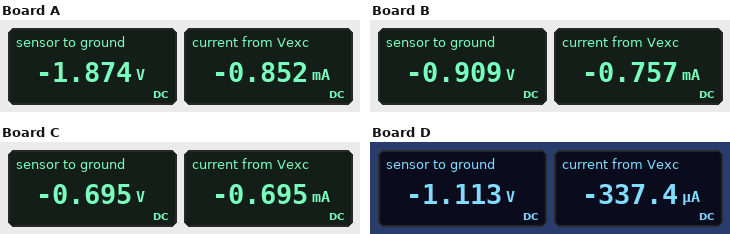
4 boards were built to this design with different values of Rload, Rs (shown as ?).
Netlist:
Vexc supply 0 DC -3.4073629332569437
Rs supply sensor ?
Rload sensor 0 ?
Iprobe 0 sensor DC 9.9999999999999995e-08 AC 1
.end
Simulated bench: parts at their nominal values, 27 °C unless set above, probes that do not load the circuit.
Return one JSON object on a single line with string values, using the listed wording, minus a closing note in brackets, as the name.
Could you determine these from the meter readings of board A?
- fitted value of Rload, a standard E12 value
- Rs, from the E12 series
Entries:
{"fitted value of Rload, a standard E12 value": "2.2 kΩ", "Rs, from the E12 series": "1.8 kΩ"}
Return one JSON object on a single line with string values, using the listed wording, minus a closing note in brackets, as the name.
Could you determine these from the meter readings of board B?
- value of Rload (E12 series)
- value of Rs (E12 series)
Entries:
{"value of Rload": "1.2 kΩ", "value of Rs": "3.3 kΩ"}
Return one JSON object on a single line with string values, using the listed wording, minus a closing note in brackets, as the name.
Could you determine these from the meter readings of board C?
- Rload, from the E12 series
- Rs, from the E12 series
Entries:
{"Rload, from the E12 series": "1 kΩ", "Rs, from the E12 series": "3.9 kΩ"}
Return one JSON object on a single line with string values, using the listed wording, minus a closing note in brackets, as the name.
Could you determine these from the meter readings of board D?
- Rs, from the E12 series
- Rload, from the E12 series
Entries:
{"Rs, from the E12 series": "6.8 kΩ", "Rload, from the E12 series": "3.3 kΩ"}
